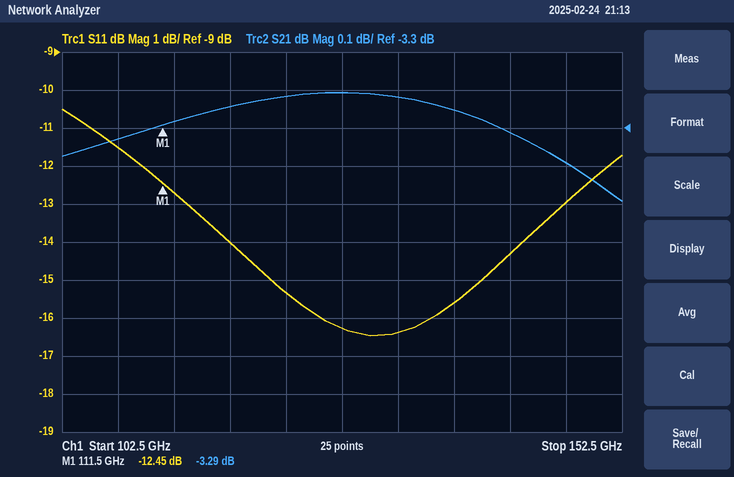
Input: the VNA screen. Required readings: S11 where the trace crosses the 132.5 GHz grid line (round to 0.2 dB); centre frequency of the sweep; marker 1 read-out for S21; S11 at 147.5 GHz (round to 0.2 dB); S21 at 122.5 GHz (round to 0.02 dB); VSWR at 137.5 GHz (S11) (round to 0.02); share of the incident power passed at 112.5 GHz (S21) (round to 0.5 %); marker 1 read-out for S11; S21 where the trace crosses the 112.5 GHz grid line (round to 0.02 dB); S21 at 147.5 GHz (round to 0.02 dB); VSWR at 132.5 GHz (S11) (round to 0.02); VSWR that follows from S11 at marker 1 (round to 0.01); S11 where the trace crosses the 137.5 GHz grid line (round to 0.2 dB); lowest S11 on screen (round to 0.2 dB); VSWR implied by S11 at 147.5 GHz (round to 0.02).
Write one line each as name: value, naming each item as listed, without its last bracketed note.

S11 where the trace crosses the 132.5 GHz grid line: -16.4 dB
centre frequency of the sweep: 127.5 GHz
marker 1 read-out for S21: -3.29 dB
S11 at 147.5 GHz: -13.0 dB
S21 at 122.5 GHz: -3.22 dB
VSWR at 137.5 GHz (S11): 1.40
share of the incident power passed at 112.5 GHz (S21): 47.0 %
marker 1 read-out for S11: -12.45 dB
S21 where the trace crosses the 112.5 GHz grid line: -3.28 dB
S21 at 147.5 GHz: -3.40 dB
VSWR at 132.5 GHz (S11): 1.36
VSWR that follows from S11 at marker 1: 1.63
S11 where the trace crosses the 137.5 GHz grid line: -15.6 dB
lowest S11 on screen: -16.4 dB
VSWR implied by S11 at 147.5 GHz: 1.58
